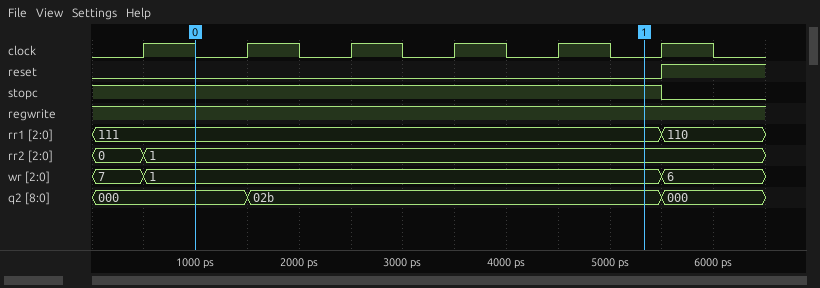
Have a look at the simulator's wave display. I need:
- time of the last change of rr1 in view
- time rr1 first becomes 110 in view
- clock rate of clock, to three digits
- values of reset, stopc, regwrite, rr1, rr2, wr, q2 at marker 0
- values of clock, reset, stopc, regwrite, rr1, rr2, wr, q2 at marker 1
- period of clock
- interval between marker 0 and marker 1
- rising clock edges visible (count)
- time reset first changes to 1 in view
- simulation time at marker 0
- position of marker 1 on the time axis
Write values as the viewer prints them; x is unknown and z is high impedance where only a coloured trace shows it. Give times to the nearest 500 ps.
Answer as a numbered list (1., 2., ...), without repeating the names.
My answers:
1. 5500 ps
2. 5500 ps
3. 1.00 GHz
4. reset=0, stopc=1, regwrite=1, rr1=111, rr2=1, wr=1, q2=000
5. clock=0, reset=0, stopc=1, regwrite=1, rr1=111, rr2=1, wr=1, q2=02b
6. 1000 ps
7. 4500 ps
8. 6
9. 5500 ps
10. 1000 ps
11. 5500 ps
